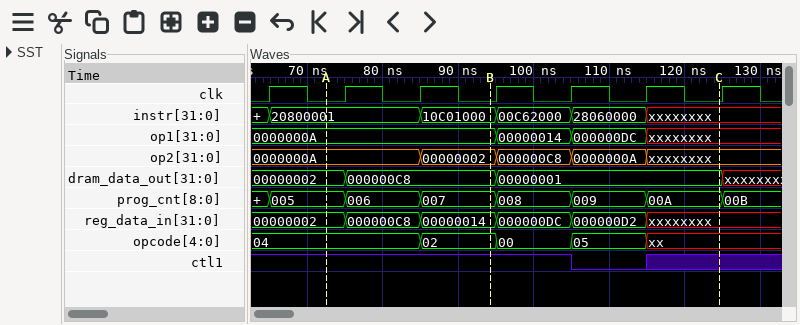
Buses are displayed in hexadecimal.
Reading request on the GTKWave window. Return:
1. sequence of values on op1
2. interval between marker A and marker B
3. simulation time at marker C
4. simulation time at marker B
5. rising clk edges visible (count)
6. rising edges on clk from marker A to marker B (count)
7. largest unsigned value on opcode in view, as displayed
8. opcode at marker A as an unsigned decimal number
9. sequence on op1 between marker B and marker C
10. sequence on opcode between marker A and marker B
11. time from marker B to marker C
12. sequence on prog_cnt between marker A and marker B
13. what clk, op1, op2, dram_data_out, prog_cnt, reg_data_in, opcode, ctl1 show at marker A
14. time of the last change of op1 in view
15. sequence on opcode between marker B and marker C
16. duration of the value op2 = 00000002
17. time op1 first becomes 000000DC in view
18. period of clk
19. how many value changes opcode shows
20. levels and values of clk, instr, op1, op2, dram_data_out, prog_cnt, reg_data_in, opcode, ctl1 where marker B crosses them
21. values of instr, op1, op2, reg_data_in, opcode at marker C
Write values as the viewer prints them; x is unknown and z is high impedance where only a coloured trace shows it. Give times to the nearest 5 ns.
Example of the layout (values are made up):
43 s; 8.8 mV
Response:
0000000A, 00000014, 000000DC, xxxxxxxx; 20 ns; 125 ns; 95 ns; 7; 2; 05; 4; 0000000A, 00000014, 000000DC, xxxxxxxx; 04, 02; 30 ns; 005, 006, 007; clk=0, op1=0000000A, op2=0000000A, dram_data_out=00000002, prog_cnt=005, reg_data_in=00000002, opcode=04, ctl1=1; 115 ns; 02, 00, 05, xx; 10 ns; 105 ns; 10 ns; 4; clk=0, instr=10C01000, op1=0000000A, op2=00000002, dram_data_out=000000C8, prog_cnt=007, reg_data_in=00000014, opcode=02, ctl1=1; instr=xxxxxxxx, op1=xxxxxxxx, op2=xxxxxxxx, reg_data_in=xxxxxxxx, opcode=xx
